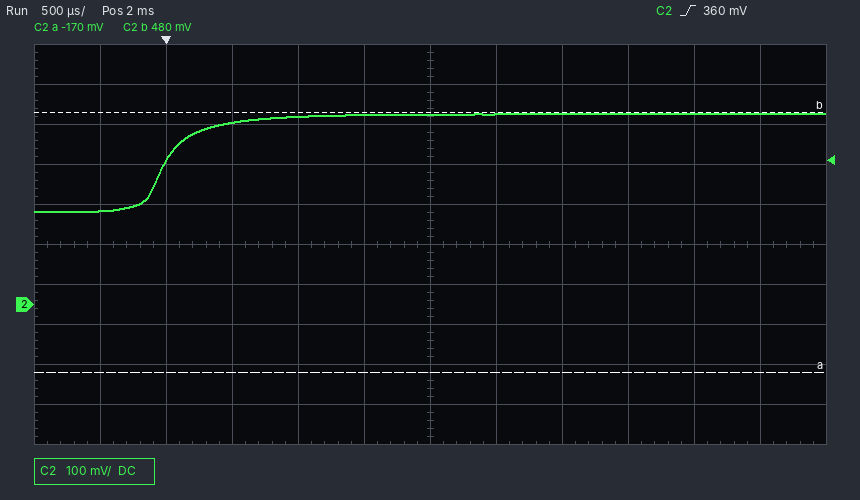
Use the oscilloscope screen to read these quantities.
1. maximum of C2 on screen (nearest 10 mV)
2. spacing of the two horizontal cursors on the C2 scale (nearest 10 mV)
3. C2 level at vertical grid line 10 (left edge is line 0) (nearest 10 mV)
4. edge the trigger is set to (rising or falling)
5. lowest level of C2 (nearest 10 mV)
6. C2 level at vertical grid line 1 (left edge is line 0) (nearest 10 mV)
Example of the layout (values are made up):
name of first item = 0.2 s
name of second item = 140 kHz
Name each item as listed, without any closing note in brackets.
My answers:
maximum of C2 on screen = 480 mV
spacing of the two horizontal cursors on the C2 scale = 650 mV
C2 level at vertical grid line 10 (left edge is line 0) = 480 mV
edge the trigger is set to = rising
lowest level of C2 = 230 mV
C2 level at vertical grid line 1 (left edge is line 0) = 230 mV
